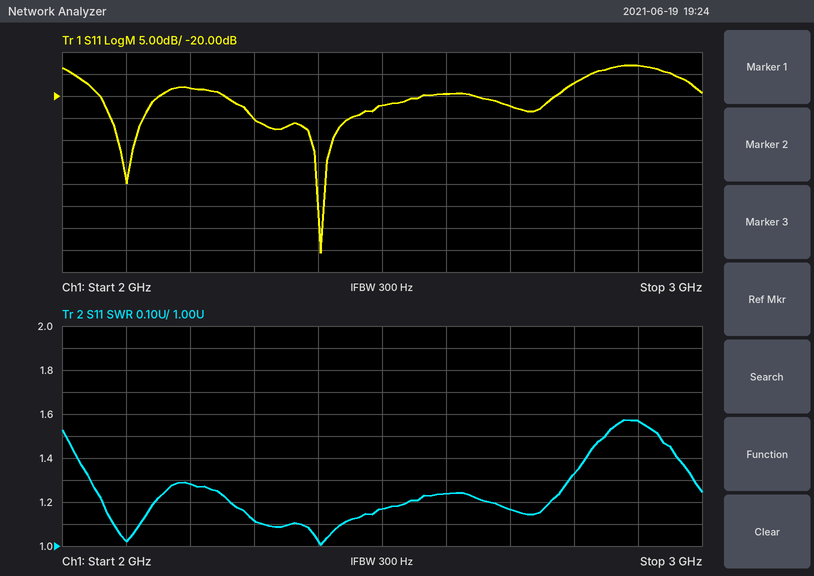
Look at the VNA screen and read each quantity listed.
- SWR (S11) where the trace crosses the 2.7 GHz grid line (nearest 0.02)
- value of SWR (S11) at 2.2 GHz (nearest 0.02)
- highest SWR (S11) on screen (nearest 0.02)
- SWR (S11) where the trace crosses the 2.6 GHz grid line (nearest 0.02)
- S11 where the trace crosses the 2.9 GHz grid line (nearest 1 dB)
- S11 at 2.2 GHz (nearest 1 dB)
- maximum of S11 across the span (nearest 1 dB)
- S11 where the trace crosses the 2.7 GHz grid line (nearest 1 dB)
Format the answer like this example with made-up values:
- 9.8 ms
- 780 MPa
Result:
- 1.16
- 1.28
- 1.58
- 1.24
- -13 dB
- -18 dB
- -13 dB
- -22 dB
